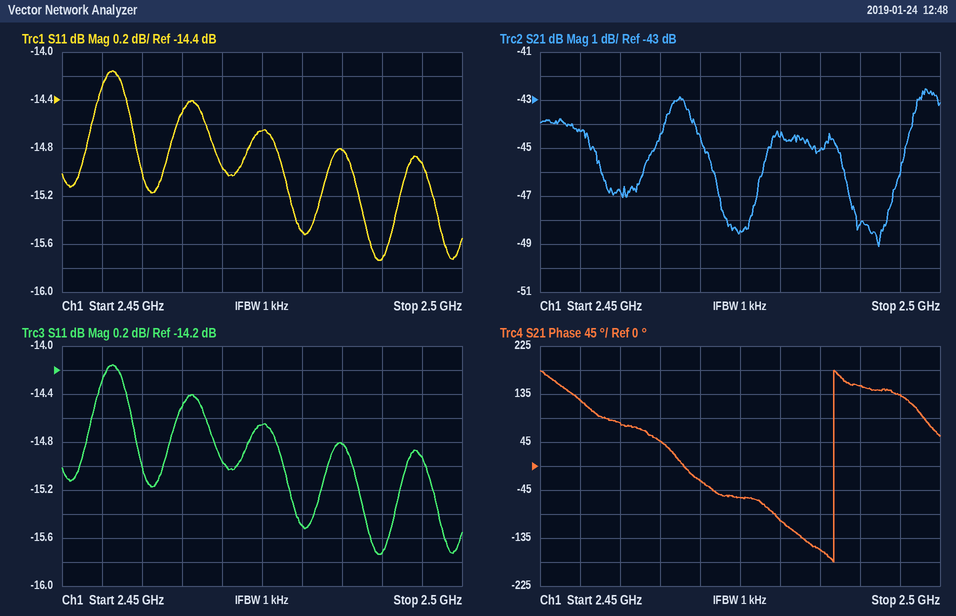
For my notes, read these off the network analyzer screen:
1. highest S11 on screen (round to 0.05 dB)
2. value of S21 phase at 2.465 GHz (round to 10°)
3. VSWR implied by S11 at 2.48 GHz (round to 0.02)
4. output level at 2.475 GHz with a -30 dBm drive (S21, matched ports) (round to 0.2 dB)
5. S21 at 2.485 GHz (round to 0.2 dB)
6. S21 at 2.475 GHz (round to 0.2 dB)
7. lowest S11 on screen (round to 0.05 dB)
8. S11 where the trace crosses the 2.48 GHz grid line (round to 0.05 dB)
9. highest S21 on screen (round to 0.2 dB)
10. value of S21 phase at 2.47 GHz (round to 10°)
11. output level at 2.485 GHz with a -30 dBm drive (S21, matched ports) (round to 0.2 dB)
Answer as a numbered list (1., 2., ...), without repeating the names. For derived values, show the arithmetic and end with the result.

1. -14.15 dB
2. 50°
3. |Γ| = 10^(-15.5/20) = 0.1679; VSWR = (1 + 0.1679)/(1 − 0.1679) ≈ 1.40
4. -30 dBm + (-48.4 dB) = -78.4 dBm
5. -45.0 dB
6. -48.4 dB
7. -15.75 dB
8. -15.50 dB
9. -42.6 dB
10. -30°
11. -30 dBm + (-45.0 dB) = -75.0 dBm
